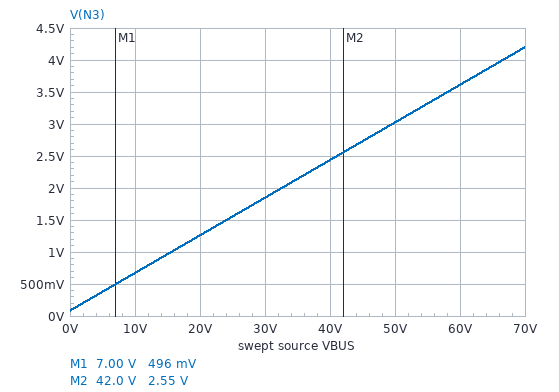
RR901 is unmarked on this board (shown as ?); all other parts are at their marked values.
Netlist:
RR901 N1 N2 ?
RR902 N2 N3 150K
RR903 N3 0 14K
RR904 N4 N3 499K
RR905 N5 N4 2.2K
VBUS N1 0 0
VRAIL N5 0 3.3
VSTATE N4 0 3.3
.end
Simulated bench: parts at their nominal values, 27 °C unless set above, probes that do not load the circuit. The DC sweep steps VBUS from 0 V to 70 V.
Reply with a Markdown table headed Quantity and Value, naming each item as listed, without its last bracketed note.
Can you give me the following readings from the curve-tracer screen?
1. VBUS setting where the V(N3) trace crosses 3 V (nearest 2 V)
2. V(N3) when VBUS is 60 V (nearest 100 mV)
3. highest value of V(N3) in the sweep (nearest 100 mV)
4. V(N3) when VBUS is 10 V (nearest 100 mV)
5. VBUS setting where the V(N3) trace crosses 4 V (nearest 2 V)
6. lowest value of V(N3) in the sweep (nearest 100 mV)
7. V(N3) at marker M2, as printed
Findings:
| Quantity | Value |
|---|---|
| VBUS setting where the V(N3) trace crosses 3 V | 50 V |
| V(N3) when VBUS is 60 V | 3.6 V |
| highest value of V(N3) in the sweep | 4.2 V |
| V(N3) when VBUS is 10 V | 700 mV |
| VBUS setting where the V(N3) trace crosses 4 V | 66 V |
| lowest value of V(N3) in the sweep | 100 mV |
| V(N3) at marker M2, as printed | 2.55 V |
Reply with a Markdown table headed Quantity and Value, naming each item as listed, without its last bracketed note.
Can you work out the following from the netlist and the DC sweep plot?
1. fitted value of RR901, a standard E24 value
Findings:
| Quantity | Value |
|---|---|
| fitted value of RR901, a standard E24 value | 68 kΩ |
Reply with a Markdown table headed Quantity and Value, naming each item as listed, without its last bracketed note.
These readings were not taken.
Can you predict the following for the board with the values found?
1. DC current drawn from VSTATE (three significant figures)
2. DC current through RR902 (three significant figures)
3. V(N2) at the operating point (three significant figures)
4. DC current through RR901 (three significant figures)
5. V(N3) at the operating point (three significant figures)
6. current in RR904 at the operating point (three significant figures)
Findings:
| Quantity | Value |
|---|---|
| DC current drawn from VSTATE | 6.44 µA |
| DC current through RR902 | 389 nA |
| V(N2) at the operating point | 26.4 mV |
| DC current through RR901 | 389 nA |
| V(N3) at the operating point | 84.8 mV |
| current in RR904 at the operating point | 6.44 µA |
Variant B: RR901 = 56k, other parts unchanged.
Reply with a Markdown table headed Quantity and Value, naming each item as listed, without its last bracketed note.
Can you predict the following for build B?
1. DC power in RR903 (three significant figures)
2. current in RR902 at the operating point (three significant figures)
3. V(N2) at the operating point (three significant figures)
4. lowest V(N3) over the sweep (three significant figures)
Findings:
| Quantity | Value |
|---|---|
| DC power in RR903 | 510 nW |
| current in RR902 at the operating point | 410 nA |
| V(N2) at the operating point | 23.0 mV |
| lowest V(N3) over the sweep | 84.5 mV |
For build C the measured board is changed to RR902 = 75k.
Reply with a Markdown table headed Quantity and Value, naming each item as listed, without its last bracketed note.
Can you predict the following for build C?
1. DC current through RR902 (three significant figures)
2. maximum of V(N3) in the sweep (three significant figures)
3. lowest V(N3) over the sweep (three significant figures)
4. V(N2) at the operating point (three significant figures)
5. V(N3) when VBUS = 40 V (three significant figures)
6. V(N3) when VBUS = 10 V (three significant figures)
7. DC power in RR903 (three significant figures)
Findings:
| Quantity | Value |
|---|---|
| DC current through RR902 | 575 nA |
| maximum of V(N3) in the sweep | 6.17 V |
| lowest V(N3) over the sweep | 82.2 mV |
| V(N2) at the operating point | 39.1 mV |
| V(N3) when VBUS = 40 V | 3.56 V |
| V(N3) when VBUS = 10 V | 952 mV |
| DC power in RR903 | 483 nW |
